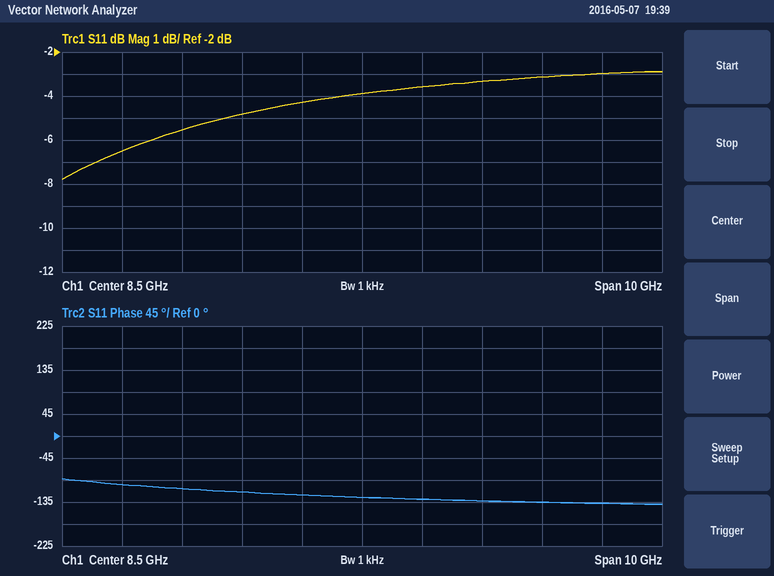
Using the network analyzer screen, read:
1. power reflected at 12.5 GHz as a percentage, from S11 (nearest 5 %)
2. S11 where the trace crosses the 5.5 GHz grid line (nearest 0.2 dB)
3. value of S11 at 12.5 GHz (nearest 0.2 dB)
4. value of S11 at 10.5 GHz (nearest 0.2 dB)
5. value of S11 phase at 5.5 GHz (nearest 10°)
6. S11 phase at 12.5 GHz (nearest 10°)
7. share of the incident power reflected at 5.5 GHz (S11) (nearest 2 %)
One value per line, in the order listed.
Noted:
50 %
-5.6 dB
-3.0 dB
-3.4 dB
-110°
-140°
28 %
